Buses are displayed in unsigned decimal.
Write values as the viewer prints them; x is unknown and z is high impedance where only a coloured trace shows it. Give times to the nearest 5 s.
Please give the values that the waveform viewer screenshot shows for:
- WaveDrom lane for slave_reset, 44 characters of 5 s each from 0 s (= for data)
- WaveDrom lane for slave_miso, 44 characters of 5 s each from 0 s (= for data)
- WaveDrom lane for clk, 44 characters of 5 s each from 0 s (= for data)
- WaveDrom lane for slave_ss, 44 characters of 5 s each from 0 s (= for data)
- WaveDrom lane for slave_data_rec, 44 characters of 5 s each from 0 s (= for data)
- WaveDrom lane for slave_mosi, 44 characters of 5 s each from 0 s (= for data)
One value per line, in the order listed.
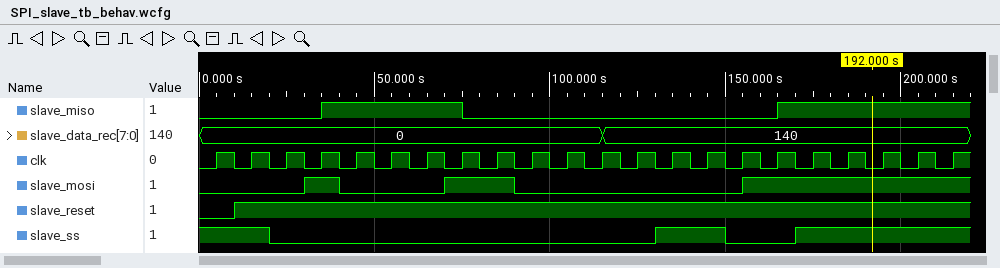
{name: 'slave_reset', wave: '0.1.........................................'}
{name: 'slave_miso', wave: '0......1.......0.................1..........'}
{name: 'clk', wave: '01010101010101010101010101010101010101010101'}
{name: 'slave_ss', wave: '1...0.....................1...0...1.........'}
{name: 'slave_data_rec', wave: '=......................=....................', data: '0 140'}
{name: 'slave_mosi', wave: '0.....1.0.....1...0............1............'}
